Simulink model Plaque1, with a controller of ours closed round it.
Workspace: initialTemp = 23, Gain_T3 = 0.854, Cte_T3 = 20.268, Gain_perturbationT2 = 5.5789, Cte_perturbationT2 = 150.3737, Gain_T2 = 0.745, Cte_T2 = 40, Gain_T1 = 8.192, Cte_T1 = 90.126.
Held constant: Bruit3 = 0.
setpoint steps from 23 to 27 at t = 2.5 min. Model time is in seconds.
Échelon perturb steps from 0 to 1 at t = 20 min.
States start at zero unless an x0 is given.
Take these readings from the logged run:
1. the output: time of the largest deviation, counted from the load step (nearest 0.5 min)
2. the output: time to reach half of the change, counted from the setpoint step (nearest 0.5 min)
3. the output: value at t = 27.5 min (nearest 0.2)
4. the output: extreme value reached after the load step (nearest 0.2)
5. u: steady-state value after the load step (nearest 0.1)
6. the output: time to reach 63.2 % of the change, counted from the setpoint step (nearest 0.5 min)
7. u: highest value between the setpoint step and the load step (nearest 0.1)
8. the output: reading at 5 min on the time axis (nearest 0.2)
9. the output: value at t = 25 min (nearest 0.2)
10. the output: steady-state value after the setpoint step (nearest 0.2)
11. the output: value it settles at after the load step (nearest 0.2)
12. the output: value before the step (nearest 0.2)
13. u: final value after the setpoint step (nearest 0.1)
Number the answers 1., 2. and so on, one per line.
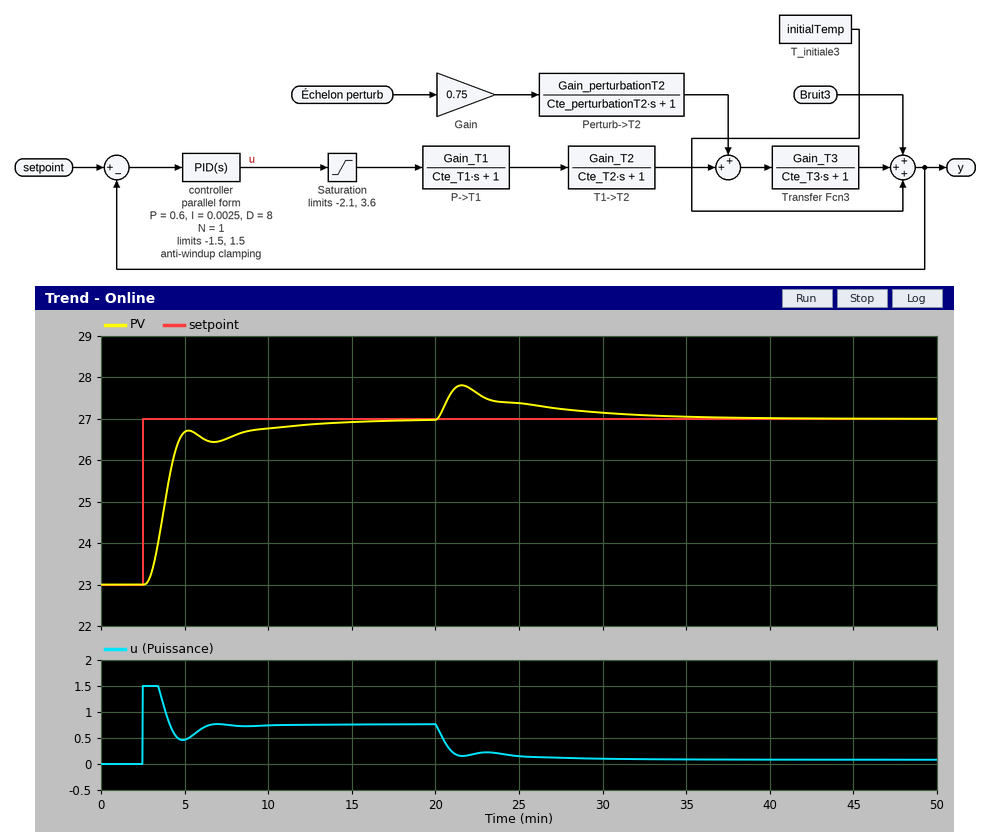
1. 1.5 min
2. 1.5 min
3. 27.2
4. 27.8
5. 0.1
6. 1.5 min
7. 1.5
8. 26.6
9. 27.4
10. 27.0
11. 27.0
12. 23.0
13. 0.8
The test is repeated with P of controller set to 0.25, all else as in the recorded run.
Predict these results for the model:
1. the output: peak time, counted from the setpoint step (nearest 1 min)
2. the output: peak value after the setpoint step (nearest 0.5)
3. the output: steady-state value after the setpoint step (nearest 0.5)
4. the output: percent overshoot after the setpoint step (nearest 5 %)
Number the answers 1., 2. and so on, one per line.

1. 5 min
2. 27.5
3. 27.0
4. 10 %
